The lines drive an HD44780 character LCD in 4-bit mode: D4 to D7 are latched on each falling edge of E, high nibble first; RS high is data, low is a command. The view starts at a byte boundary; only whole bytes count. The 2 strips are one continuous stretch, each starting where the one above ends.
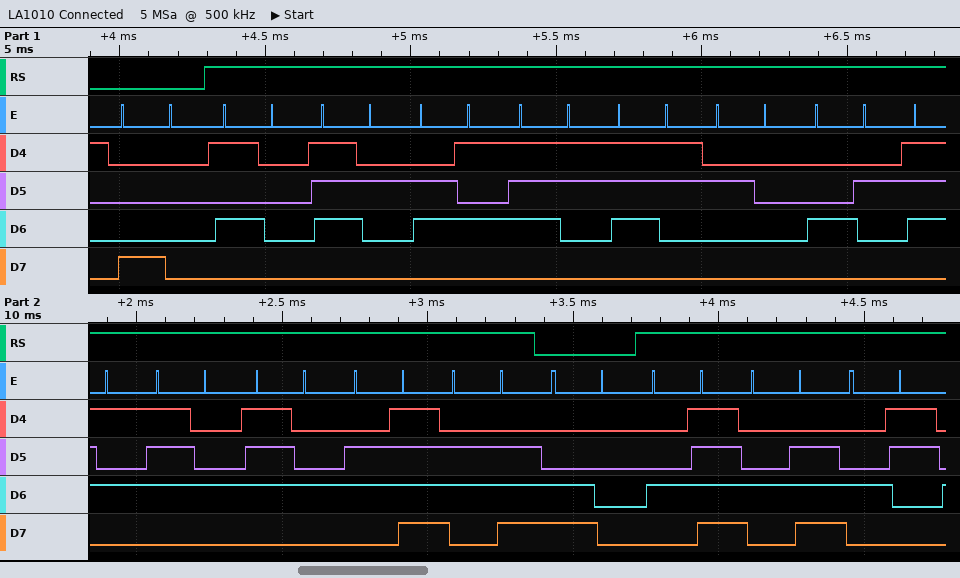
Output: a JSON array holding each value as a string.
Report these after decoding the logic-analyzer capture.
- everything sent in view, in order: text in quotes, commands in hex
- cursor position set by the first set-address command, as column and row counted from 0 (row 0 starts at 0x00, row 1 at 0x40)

["0x80 \"Press Button\" 0xC0 \"ONC\"", "column 0, row 0"]
